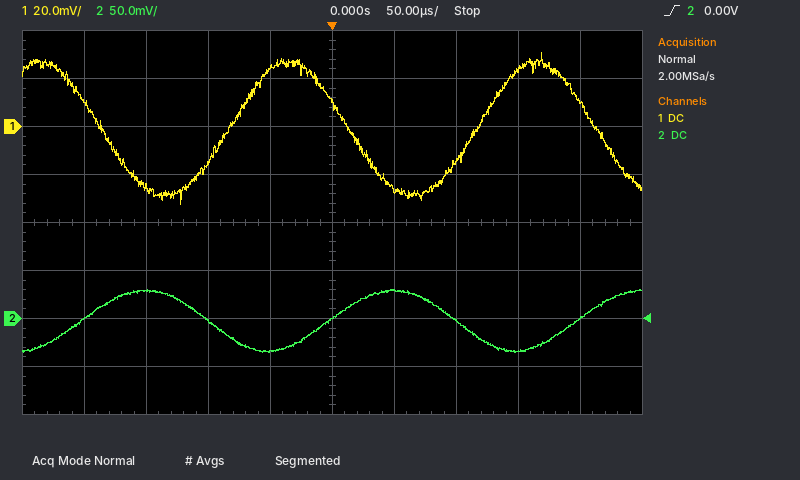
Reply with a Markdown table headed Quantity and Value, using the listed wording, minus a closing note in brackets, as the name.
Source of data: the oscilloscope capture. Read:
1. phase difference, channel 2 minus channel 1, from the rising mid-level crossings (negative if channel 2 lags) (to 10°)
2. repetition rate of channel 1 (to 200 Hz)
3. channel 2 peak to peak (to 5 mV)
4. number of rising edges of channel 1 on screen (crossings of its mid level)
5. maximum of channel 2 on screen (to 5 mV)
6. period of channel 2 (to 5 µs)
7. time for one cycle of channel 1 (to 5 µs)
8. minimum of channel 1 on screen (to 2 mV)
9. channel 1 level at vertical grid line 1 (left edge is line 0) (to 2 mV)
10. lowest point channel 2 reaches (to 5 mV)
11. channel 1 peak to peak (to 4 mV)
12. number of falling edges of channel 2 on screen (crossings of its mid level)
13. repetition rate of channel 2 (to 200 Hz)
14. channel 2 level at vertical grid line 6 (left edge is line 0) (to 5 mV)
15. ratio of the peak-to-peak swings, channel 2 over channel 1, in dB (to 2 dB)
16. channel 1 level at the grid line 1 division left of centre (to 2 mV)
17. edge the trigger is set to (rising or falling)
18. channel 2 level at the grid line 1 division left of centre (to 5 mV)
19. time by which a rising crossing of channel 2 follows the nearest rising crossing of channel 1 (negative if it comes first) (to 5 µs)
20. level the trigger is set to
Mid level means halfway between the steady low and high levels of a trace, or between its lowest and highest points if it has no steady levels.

| Quantity | Value |
|---|---|
| phase difference, channel 2 minus channel 1, from the rising mid-level crossings (negative if channel 2 lags) | -140° |
| repetition rate of channel 1 | 5.0 kHz |
| channel 2 peak to peak | 65 mV |
| number of rising edges of channel 1 on screen | 2 |
| maximum of channel 2 on screen | 30 mV |
| period of channel 2 | 200 µs |
| time for one cycle of channel 1 | 200 µs |
| minimum of channel 1 on screen | -32 mV |
| channel 1 level at vertical grid line 1 (left edge is line 0) | 10 mV |
| lowest point channel 2 reaches | -35 mV |
| channel 1 peak to peak | 64 mV |
| number of falling edges of channel 2 on screen | 2 |
| repetition rate of channel 2 | 5.0 kHz |
| channel 2 level at vertical grid line 6 (left edge is line 0) | 30 mV |
| ratio of the peak-to-peak swings, channel 2 over channel 1, in dB | 0 dB |
| channel 1 level at the grid line 1 division left of centre | 24 mV |
| edge the trigger is set to | rising |
| channel 2 level at the grid line 1 division left of centre | -35 mV |
| time by which a rising crossing of channel 2 follows the nearest rising crossing of channel 1 (negative if it comes first) | +80 µs |
| level the trigger is set to | 0.00 V |
